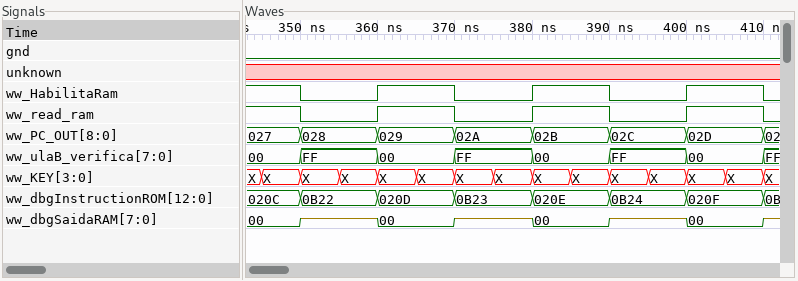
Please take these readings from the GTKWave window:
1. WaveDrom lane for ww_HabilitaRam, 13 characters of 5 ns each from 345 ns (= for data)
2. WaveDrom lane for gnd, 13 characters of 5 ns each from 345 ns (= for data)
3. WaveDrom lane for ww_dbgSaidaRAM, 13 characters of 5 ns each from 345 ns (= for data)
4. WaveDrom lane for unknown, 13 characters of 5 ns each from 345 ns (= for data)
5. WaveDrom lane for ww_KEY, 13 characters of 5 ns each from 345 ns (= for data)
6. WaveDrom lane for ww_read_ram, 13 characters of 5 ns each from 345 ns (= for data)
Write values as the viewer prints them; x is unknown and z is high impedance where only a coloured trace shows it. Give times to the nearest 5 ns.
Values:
{name: 'ww_HabilitaRam', wave: '10.1.0.1.0.1.'}
{name: 'gnd', wave: '0............'}
{name: 'ww_dbgSaidaRAM', wave: '=z.=.z.=.z.=.', data: '00 00 00 00'}
{name: 'unknown', wave: 'x............'}
{name: 'ww_KEY', wave: '=============', data: 'X X X X X X X X X X X X X'}
{name: 'ww_read_ram', wave: '10.1.0.1.0.1.'}
